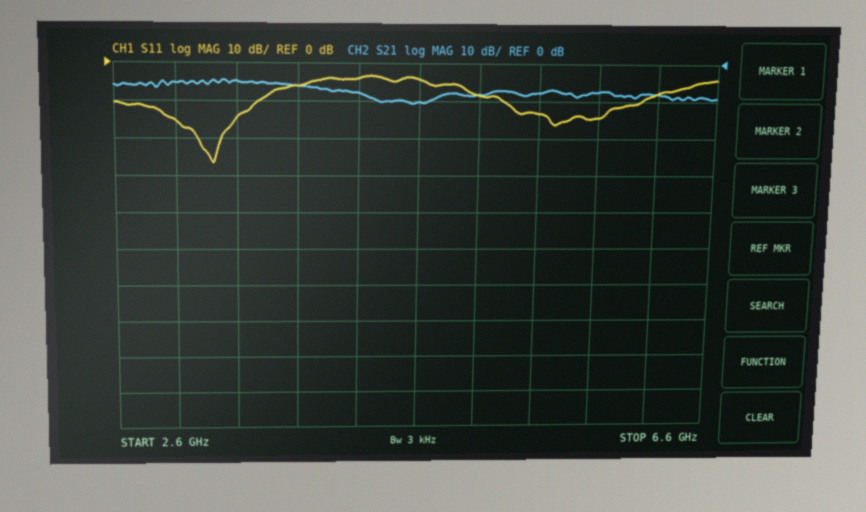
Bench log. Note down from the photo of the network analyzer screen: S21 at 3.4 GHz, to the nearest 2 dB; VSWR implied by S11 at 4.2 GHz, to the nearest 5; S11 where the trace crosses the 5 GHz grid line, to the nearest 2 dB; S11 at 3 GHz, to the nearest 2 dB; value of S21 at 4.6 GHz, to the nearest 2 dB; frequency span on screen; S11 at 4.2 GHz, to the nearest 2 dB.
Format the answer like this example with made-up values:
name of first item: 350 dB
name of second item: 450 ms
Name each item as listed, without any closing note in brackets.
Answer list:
S21 at 3.4 GHz, to the nearest 2 dB: -4 dB
VSWR implied by S11 at 4.2 GHz, to the nearest 5: 5
S11 where the trace crosses the 5 GHz grid line, to the nearest 2 dB: -8 dB
S11 at 3 GHz, to the nearest 2 dB: -16 dB
value of S21 at 4.6 GHz, to the nearest 2 dB: -10 dB
frequency span on screen: 4 GHz
S11 at 4.2 GHz, to the nearest 2 dB: -4 dB
